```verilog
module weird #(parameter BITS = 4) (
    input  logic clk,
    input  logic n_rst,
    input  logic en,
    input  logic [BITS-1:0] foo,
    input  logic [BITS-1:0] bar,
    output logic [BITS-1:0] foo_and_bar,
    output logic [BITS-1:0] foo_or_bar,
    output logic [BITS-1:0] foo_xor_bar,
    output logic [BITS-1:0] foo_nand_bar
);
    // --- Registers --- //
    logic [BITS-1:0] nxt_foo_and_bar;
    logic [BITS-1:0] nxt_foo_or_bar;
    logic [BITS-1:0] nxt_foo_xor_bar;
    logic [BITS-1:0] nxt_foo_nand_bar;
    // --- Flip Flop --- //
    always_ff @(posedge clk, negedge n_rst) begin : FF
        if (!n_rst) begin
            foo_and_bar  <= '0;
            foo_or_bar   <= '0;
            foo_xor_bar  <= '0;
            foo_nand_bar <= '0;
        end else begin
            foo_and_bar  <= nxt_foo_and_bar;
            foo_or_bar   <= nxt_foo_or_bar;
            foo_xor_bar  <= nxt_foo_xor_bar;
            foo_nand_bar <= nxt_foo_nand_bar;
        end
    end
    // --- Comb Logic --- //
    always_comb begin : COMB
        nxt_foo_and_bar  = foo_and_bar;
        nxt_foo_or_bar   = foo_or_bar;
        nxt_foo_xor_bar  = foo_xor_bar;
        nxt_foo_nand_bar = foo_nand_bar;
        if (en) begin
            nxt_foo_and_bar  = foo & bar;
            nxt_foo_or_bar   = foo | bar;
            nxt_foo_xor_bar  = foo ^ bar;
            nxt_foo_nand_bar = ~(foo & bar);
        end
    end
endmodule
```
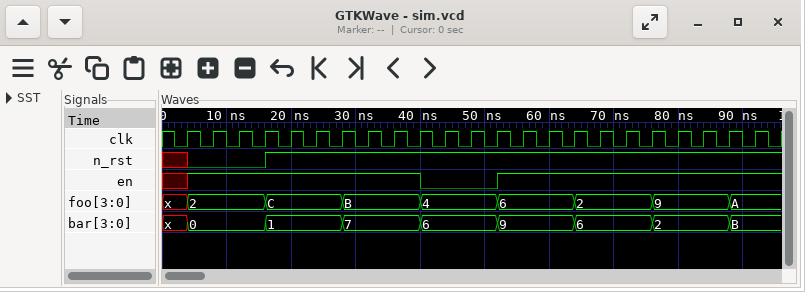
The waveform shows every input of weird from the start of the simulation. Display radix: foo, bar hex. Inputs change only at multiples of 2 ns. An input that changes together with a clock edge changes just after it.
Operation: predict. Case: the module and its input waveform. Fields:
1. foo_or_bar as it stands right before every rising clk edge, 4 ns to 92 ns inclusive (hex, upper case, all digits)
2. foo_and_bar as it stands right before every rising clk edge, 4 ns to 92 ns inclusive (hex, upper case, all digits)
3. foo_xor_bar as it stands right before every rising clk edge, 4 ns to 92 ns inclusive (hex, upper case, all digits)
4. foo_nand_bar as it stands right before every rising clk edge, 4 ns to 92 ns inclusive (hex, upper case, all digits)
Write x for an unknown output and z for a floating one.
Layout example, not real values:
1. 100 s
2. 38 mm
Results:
1. x, 0, 0, 0, 0, D, D, D, F, F, F, F, F, F, F, F, F, 6, 6, 6, B, B, B
2. x, 0, 0, 0, 0, 0, 0, 0, 3, 3, 3, 3, 3, 3, 0, 0, 0, 2, 2, 2, 0, 0, 0
3. x, 0, 0, 0, 0, D, D, D, C, C, C, C, C, C, F, F, F, 4, 4, 4, B, B, B
4. x, 0, 0, 0, 0, F, F, F, C, C, C, C, C, C, F, F, F, D, D, D, F, F, F
